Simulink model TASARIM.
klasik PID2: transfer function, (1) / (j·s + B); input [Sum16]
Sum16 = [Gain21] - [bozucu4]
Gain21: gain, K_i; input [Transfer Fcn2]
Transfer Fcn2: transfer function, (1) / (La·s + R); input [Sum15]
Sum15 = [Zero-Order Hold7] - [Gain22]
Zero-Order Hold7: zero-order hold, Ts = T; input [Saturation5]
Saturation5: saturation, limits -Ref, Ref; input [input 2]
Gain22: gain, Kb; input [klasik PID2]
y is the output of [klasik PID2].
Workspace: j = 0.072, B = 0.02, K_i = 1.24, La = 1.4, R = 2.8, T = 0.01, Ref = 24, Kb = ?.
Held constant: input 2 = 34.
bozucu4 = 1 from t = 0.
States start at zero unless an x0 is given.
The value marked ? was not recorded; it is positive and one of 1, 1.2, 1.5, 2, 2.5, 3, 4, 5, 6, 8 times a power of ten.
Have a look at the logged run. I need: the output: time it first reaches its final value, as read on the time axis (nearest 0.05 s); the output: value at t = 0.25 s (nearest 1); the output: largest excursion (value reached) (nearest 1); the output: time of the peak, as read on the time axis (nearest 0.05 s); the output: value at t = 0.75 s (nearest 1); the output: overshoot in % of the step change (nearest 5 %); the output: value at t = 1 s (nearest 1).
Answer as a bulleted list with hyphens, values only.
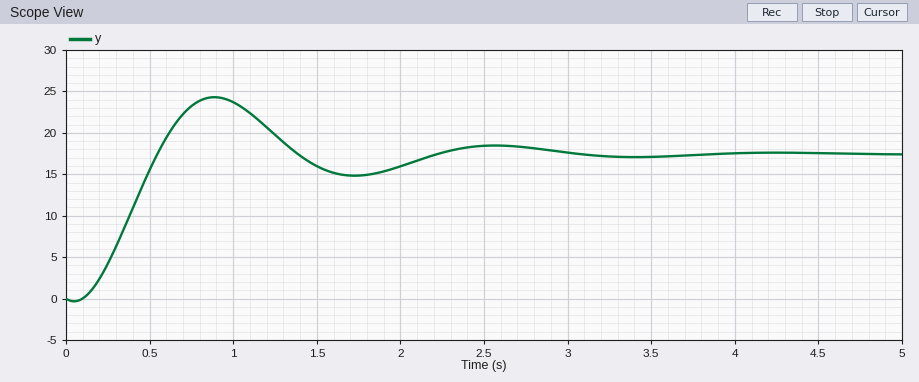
- 0.55 s
- 4
- 24
- 0.90 s
- 23
- 40 %
- 24
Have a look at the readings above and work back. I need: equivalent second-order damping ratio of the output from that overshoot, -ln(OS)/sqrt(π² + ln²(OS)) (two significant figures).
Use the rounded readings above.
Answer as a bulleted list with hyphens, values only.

- 0.28
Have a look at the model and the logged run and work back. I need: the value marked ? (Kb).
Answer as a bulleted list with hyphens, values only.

- 1.2
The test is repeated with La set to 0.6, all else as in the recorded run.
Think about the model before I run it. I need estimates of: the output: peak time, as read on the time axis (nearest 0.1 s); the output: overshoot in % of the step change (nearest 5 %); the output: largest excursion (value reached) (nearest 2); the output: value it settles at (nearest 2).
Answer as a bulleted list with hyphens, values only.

- 0.6 s
- 25 %
- 22
- 18
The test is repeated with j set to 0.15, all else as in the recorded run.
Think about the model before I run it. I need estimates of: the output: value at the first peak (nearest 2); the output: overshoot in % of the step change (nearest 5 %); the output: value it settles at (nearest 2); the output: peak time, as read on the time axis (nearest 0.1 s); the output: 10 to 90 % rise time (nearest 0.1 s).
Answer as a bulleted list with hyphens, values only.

- 22
- 25 %
- 18
- 1.3 s
- 0.5 s
